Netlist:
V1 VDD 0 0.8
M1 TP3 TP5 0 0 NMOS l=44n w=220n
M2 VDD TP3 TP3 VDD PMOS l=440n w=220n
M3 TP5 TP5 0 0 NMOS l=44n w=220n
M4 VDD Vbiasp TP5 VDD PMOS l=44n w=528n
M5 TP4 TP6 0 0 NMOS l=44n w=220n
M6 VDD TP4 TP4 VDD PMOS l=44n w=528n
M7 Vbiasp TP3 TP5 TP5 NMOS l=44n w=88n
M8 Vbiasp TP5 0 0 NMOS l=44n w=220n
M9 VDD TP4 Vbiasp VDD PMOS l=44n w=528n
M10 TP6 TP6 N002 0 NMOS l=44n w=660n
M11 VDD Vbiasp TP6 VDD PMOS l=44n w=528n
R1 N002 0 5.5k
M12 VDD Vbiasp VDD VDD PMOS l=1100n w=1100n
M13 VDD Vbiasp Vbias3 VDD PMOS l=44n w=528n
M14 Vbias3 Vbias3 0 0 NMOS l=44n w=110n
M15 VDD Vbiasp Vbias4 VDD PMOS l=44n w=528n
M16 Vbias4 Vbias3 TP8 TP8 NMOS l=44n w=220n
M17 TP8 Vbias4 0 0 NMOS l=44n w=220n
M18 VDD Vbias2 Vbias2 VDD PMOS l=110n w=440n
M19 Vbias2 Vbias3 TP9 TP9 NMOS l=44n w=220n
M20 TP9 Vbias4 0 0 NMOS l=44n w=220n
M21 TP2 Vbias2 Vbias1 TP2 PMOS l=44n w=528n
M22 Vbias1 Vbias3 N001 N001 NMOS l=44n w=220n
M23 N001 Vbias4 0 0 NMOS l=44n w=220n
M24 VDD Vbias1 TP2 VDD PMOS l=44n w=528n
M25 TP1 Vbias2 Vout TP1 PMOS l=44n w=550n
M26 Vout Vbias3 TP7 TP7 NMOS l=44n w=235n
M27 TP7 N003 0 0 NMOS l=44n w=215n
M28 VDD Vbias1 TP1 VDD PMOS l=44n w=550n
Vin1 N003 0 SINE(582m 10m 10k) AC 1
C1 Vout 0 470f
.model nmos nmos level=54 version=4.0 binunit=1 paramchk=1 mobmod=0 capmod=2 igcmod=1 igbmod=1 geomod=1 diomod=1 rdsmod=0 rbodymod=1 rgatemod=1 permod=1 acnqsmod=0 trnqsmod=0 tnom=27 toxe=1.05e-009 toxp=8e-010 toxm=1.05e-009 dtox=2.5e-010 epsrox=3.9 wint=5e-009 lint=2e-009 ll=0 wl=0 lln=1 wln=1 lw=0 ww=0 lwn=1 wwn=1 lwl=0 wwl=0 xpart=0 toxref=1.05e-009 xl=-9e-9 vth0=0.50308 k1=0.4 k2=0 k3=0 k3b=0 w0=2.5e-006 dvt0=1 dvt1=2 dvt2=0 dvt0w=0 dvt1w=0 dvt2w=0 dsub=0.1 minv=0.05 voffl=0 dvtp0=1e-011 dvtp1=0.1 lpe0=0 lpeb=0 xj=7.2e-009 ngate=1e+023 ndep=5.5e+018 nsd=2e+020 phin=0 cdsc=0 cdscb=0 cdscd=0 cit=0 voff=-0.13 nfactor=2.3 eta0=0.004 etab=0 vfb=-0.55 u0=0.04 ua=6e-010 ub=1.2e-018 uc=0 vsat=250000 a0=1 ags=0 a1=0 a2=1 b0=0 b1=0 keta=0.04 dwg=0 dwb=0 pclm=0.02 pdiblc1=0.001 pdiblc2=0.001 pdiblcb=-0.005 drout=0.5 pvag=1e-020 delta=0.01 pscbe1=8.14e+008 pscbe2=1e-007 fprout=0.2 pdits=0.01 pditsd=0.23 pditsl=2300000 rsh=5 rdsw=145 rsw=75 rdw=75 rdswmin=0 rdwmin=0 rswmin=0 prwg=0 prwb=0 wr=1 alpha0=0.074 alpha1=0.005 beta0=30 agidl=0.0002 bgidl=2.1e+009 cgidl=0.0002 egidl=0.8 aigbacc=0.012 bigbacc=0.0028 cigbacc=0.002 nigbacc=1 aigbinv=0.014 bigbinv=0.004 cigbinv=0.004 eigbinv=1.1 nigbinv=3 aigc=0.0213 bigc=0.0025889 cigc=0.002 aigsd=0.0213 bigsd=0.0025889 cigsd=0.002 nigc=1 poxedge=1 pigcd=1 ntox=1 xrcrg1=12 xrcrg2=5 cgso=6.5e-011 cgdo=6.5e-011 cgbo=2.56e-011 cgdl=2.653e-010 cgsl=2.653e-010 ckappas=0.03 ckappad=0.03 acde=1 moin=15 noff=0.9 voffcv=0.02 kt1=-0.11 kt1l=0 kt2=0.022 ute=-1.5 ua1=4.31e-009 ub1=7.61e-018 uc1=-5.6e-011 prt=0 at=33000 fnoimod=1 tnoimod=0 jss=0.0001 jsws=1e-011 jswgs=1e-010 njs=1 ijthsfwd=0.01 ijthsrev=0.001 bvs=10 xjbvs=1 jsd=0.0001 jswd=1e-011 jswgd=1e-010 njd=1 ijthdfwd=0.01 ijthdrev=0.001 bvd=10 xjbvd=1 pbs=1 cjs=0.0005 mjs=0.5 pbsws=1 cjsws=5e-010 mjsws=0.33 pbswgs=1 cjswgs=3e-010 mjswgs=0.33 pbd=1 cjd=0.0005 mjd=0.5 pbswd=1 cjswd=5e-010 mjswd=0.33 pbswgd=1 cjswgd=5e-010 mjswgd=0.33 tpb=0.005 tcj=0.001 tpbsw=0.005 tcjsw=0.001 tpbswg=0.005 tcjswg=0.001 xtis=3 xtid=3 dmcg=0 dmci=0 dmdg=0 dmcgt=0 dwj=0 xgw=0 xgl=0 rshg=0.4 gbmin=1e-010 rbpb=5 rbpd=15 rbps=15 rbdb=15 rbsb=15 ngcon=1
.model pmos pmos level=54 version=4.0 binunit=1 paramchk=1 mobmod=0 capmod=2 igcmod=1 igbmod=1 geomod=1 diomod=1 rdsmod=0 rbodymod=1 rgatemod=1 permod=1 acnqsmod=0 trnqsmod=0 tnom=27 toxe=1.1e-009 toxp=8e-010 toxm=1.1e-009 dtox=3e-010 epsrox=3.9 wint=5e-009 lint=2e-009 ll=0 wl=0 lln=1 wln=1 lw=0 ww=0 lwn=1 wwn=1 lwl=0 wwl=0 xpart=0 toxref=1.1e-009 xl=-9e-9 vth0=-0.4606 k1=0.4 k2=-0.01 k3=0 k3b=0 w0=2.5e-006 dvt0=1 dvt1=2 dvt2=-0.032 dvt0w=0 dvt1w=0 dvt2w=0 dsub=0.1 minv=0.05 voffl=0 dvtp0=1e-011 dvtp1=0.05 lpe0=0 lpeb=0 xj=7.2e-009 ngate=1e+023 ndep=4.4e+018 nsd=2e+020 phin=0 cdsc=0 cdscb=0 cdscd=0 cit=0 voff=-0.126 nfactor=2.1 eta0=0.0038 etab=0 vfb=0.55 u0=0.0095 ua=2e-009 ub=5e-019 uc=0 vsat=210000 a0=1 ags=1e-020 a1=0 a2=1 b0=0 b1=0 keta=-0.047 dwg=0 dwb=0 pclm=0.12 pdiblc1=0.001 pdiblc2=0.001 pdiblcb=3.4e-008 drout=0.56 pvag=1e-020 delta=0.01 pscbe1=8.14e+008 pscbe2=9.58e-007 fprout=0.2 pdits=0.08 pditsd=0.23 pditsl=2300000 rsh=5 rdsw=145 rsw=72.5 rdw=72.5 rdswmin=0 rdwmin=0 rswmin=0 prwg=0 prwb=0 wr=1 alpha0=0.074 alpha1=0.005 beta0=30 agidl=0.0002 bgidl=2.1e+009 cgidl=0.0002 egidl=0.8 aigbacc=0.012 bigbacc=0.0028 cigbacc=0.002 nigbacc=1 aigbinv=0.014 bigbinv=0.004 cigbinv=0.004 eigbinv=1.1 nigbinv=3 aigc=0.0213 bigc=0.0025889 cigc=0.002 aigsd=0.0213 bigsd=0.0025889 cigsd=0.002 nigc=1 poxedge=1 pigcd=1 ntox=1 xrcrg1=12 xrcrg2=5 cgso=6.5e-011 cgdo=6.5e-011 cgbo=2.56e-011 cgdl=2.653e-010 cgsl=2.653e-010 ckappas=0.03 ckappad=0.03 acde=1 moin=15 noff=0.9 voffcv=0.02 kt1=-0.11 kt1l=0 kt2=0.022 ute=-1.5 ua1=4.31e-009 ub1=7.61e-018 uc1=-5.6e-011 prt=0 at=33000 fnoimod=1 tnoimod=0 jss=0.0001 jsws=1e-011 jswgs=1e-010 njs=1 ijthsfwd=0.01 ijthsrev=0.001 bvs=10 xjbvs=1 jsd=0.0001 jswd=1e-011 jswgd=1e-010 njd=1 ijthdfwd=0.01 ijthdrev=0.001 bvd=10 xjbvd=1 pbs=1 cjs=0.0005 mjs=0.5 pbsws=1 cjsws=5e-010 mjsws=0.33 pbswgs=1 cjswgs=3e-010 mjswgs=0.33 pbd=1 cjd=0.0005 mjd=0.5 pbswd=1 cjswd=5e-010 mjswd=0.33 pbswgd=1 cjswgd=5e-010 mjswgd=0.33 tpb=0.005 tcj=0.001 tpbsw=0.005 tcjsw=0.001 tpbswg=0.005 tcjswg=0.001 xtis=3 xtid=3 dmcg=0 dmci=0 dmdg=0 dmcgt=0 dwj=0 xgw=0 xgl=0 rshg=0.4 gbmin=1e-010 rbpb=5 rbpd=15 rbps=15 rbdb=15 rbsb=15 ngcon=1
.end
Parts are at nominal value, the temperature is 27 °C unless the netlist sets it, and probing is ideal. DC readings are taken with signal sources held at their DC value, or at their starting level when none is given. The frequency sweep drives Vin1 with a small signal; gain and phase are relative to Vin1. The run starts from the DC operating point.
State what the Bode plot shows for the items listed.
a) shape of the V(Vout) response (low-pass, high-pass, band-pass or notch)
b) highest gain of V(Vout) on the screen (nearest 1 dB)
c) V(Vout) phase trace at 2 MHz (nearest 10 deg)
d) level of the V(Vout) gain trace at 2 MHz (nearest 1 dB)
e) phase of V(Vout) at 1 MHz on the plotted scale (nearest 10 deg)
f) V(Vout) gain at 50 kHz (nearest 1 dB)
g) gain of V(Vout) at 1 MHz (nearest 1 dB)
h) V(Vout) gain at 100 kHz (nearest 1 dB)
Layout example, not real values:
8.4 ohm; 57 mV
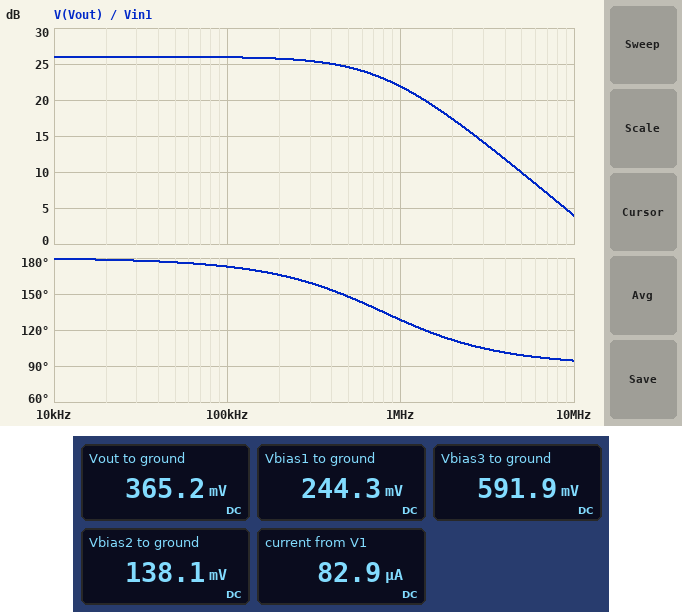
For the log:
low-pass; 26 dB; 110 deg; 17 dB; 130 deg; 26 dB; 22 dB; 26 dB
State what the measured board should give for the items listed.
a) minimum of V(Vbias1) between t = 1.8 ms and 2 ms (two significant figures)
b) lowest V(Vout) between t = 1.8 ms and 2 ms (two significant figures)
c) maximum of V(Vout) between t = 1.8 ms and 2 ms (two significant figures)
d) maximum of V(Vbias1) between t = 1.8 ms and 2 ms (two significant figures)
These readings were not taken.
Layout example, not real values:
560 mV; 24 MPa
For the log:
240 mV; 210 mV; 550 mV; 240 mV
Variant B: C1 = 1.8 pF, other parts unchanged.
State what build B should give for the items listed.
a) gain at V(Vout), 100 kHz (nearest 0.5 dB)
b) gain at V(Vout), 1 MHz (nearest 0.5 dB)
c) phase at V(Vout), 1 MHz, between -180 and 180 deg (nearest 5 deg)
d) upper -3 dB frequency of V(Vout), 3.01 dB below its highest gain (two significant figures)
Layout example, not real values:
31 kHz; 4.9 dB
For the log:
25.0 dB; 12.0 dB; 100 deg; 210 kHz
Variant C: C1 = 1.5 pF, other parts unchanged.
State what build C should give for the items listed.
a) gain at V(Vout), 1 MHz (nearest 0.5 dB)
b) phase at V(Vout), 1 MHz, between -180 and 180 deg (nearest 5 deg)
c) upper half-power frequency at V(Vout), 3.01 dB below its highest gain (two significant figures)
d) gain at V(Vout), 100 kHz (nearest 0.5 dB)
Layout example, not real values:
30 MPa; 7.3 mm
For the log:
13.5 dB; 105 deg; 250 kHz; 25.5 dB
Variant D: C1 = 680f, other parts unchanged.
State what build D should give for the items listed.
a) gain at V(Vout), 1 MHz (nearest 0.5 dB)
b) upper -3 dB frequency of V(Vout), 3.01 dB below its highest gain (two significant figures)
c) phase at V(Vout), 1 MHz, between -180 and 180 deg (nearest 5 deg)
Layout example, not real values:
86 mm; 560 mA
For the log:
19.5 dB; 550 kHz; 120 deg
